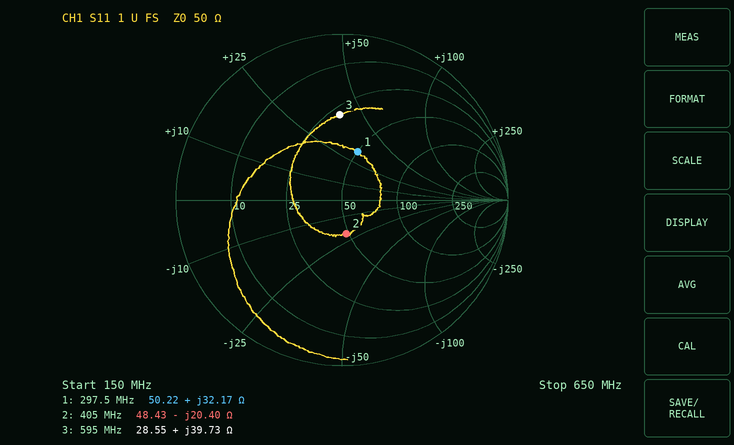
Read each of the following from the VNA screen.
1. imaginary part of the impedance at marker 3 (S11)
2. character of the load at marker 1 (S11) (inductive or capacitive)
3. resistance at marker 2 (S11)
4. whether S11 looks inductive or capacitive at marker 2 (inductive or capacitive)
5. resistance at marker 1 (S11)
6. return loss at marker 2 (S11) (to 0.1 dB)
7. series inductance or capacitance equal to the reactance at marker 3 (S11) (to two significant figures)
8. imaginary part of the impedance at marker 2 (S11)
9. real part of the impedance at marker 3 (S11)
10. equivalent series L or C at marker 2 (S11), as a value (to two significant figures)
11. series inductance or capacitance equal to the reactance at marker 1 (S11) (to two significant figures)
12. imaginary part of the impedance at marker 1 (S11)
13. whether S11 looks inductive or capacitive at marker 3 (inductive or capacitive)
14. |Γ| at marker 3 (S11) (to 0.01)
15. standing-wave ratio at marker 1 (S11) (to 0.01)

+39.73 Ω
inductive
48.43 Ω
capacitive
50.22 Ω
13.8 dB
11 nH
-20.40 Ω
28.55 Ω
19 pF
17 nH
+32.17 Ω
inductive
0.51
1.88
